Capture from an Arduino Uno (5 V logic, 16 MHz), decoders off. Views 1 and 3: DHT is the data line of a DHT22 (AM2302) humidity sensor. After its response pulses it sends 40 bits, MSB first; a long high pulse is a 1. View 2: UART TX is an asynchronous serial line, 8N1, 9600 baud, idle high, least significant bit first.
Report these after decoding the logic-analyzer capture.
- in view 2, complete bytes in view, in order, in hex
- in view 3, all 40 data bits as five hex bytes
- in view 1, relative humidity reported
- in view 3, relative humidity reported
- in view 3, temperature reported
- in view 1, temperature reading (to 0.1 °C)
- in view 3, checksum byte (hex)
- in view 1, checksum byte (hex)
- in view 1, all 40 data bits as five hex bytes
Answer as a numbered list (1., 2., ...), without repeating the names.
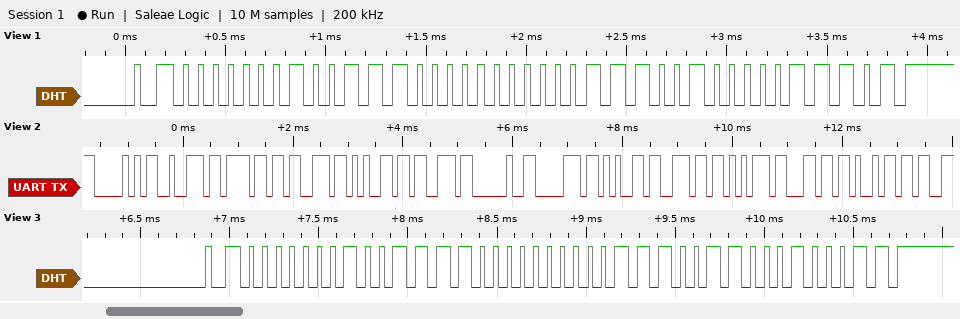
1. 50 72 6F 73 65 73 20 70 65 6E 75 6C 69
2. 01 3C 00 E6 23
3. 31.2 %
4. 31.6 %
5. 23.0 °C
6. 22.8 °C
7. 0x23
8. 0x1D
9. 01 38 00 E4 1D
